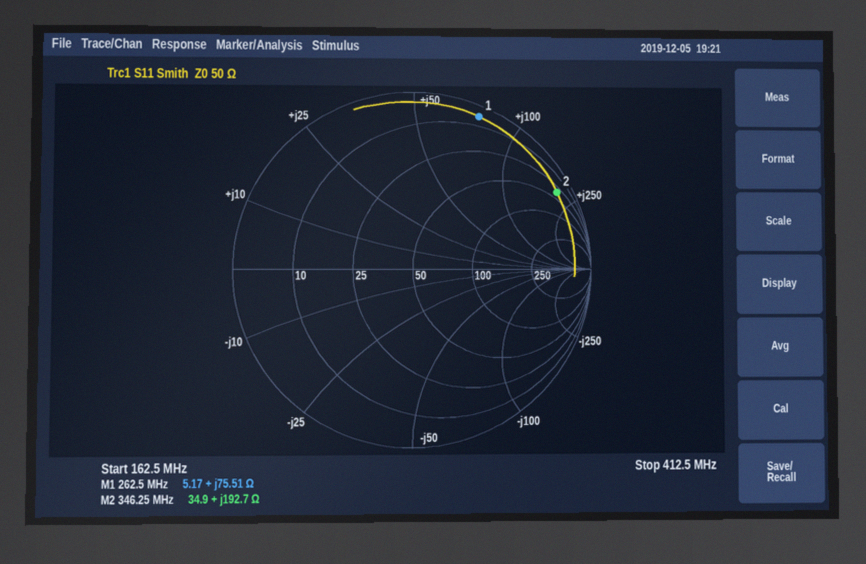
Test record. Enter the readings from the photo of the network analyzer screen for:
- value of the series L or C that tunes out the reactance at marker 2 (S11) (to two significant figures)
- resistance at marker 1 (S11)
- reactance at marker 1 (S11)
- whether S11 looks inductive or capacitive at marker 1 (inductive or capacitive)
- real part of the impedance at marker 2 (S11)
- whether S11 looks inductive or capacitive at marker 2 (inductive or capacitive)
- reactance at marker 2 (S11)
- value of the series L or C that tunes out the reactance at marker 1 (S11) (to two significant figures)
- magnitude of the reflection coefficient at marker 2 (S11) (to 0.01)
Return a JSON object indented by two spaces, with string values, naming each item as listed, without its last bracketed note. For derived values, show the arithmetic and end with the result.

{
  "value of the series L or C that tunes out the reactance at marker 2 (S11)": "C = 1/(2π × 346.25 MHz × 192.7 Ω) ≈ 2.4 pF",
  "resistance at marker 1": "5.17 Ω",
  "reactance at marker 1": "+75.51 Ω",
  "whether S11 looks inductive or capacitive at marker 1": "inductive",
  "real part of the impedance at marker 2": "34.9 Ω",
  "whether S11 looks inductive or capacitive at marker 2": "inductive",
  "reactance at marker 2": "+192.7 Ω",
  "value of the series L or C that tunes out the reactance at marker 1 (S11)": "C = 1/(2π × 262.5 MHz × 75.51 Ω) ≈ 8.0 pF",
  "magnitude of the reflection coefficient at marker 2 (S11)": "0.92"
}
